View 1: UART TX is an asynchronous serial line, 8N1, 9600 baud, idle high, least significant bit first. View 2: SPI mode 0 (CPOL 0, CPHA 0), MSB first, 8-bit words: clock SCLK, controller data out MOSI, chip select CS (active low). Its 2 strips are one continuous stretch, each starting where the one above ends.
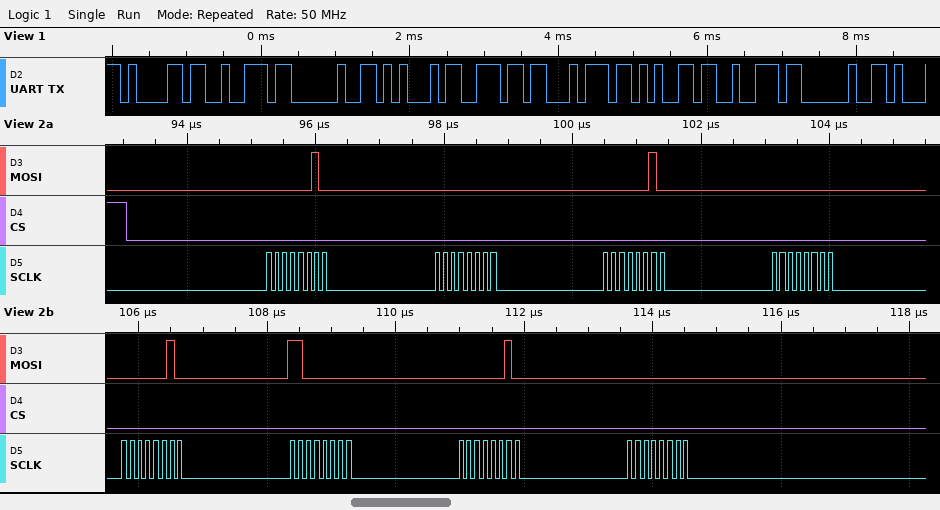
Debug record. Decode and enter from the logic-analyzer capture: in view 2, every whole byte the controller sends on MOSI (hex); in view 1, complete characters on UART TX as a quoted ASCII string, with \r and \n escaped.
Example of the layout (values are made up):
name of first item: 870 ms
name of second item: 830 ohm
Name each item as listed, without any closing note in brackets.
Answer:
in view 2, every whole byte the controller sends on MOSI: 02 00 02 00 02 C0 02 00
in view 1, complete characters on UART TX as a quoted ASCII string, with \r and \n escaped: "ar Enter "
